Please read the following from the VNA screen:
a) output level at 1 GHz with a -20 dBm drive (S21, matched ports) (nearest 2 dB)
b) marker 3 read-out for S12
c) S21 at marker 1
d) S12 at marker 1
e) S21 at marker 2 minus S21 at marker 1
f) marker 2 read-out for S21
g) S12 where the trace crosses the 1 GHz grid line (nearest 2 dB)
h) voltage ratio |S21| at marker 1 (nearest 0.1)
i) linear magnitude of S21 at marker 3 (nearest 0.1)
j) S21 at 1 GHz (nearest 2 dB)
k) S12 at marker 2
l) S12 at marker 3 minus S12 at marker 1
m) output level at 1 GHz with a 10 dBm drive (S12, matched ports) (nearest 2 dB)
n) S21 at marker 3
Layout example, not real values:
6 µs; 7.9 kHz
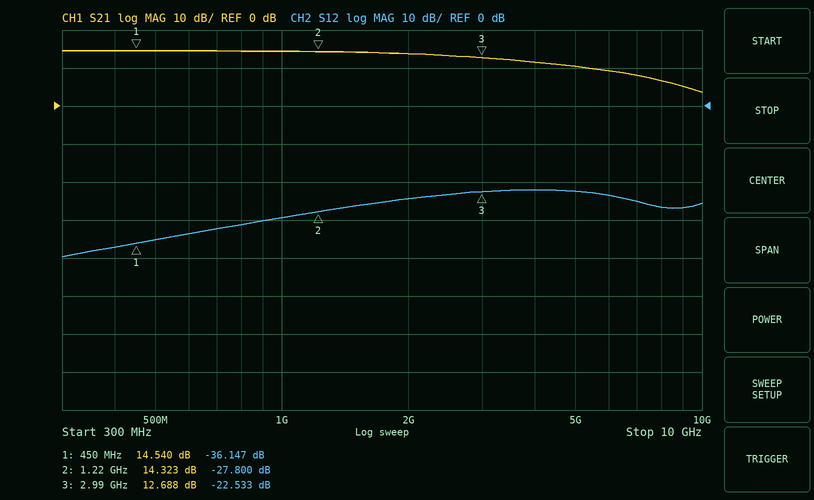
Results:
-6 dBm; -22.533 dB; 14.540 dB; -36.147 dB; -0.217 dB; 14.323 dB; -30 dB; 5.3; 4.3; 14 dB; -27.800 dB; 13.614 dB; -20 dBm; 12.688 dB
